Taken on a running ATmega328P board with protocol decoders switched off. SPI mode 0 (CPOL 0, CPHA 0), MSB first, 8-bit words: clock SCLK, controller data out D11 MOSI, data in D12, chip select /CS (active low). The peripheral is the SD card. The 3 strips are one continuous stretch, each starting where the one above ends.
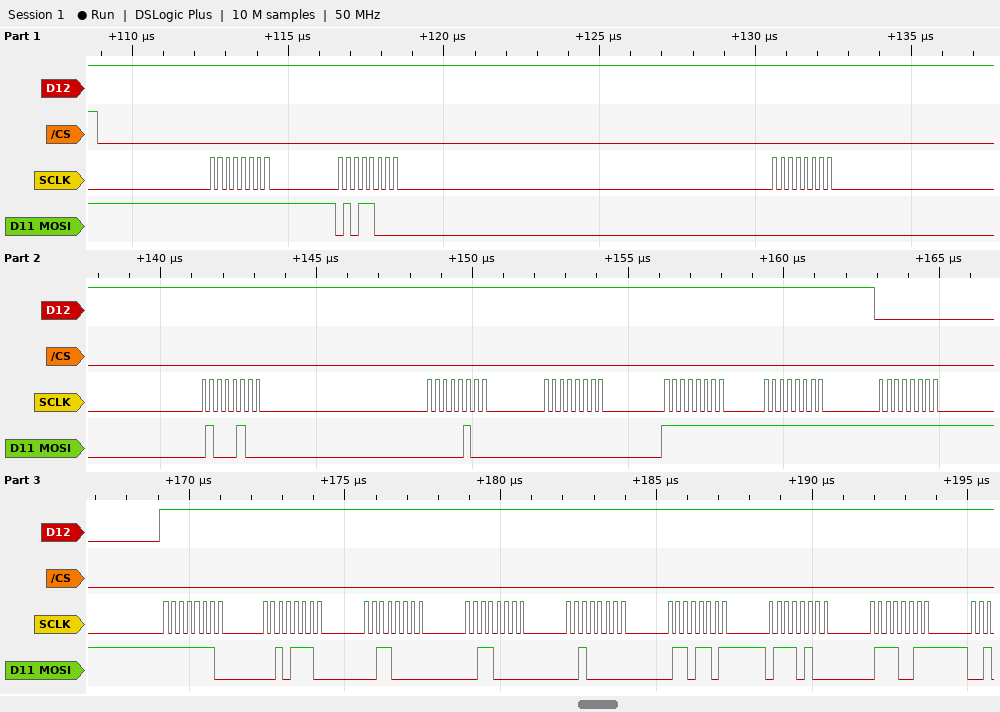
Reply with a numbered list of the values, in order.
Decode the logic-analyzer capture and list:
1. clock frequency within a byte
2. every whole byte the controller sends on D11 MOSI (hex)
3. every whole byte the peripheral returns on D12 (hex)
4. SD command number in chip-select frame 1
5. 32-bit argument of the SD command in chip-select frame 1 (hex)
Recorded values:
1. 4 MHz
2. 0xFF 0x58 0x00 0x44 0x04 0x00 0xFF 0xFF 0xFF 0xFE 0x2E 0x30 0x30 0x20 0x6D 0x74 0x73
3. 0xFF 0xFF 0xFF 0xFF 0xFF 0xFF 0xFF 0xFF 0x00 0xFF 0xFF 0xFF 0xFF 0xFF 0xFF 0xFF 0xFF
4. CMD24
5. 0x00440400
